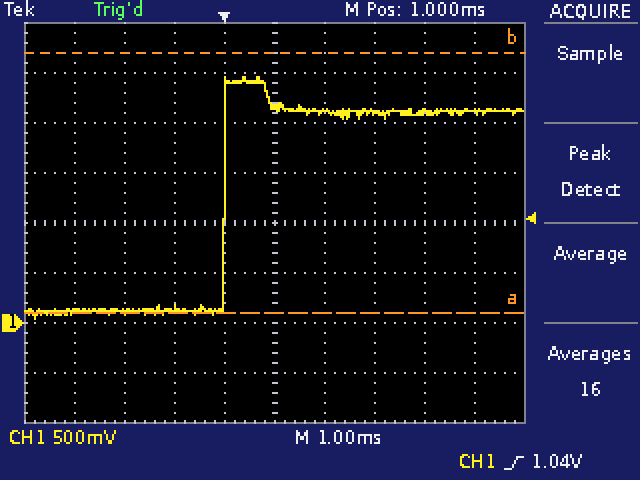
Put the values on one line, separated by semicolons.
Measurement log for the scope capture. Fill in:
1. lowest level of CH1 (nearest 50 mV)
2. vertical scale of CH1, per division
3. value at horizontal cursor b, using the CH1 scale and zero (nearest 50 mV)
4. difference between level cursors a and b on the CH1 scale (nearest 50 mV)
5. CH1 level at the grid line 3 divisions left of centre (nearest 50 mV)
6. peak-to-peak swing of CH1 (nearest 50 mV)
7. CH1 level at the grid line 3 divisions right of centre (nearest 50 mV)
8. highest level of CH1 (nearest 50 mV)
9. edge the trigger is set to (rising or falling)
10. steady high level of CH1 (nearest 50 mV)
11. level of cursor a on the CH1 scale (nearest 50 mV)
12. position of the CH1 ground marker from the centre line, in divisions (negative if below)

50 mV; 500 mV; 2.70 V; 2.60 V; 100 mV; 2.40 V; 2.10 V; 2.45 V; rising; 2.10 V; 100 mV; -2.0 div
